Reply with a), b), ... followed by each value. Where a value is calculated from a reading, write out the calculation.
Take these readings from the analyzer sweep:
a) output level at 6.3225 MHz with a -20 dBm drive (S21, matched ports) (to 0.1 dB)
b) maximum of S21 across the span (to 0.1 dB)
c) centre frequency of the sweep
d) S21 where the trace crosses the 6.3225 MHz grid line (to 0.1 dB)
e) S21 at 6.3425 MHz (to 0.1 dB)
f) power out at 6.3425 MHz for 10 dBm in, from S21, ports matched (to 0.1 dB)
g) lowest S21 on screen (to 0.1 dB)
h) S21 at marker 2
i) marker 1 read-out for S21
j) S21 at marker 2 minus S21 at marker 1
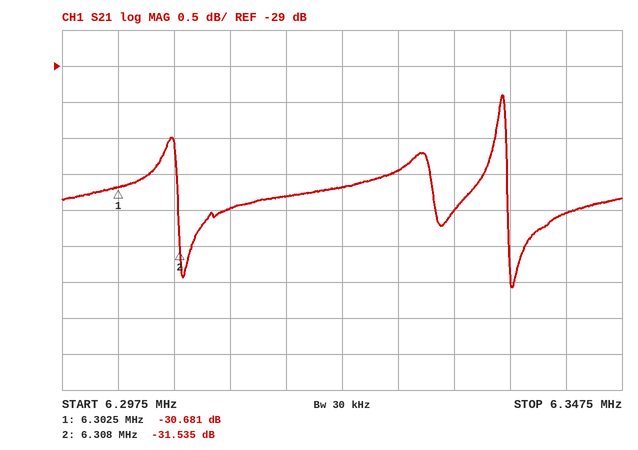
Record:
a) -20 dBm + (-30.7 dB) = -50.7 dBm
b) -29.4 dB
c) 6.3225 MHz
d) -30.7 dB
e) -31.0 dB
f) 10 dBm + (-31.0 dB) = -21.0 dBm
g) -32.1 dB
h) -31.535 dB
i) -30.681 dB
j) -31.535 − (-30.681) = -0.854 dB
